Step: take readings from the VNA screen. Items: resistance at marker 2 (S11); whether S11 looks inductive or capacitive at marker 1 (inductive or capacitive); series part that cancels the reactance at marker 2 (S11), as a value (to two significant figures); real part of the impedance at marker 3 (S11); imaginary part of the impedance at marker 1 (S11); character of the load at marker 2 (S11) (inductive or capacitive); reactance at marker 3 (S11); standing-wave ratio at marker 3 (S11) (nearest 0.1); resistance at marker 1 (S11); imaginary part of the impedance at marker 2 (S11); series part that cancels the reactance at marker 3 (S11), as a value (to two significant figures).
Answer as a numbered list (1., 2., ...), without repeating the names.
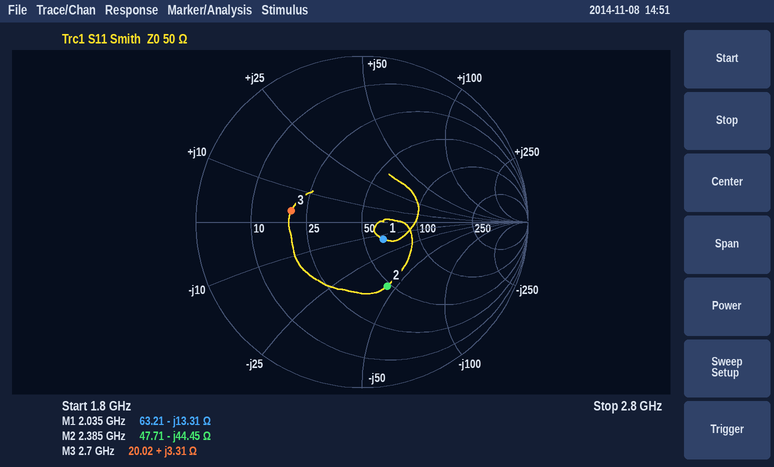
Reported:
1. 47.71 Ω
2. capacitive
3. 3.0 nH
4. 20.02 Ω
5. -13.31 Ω
6. capacitive
7. +3.31 Ω
8. 2.5
9. 63.21 Ω
10. -44.45 Ω
11. 18 pF
